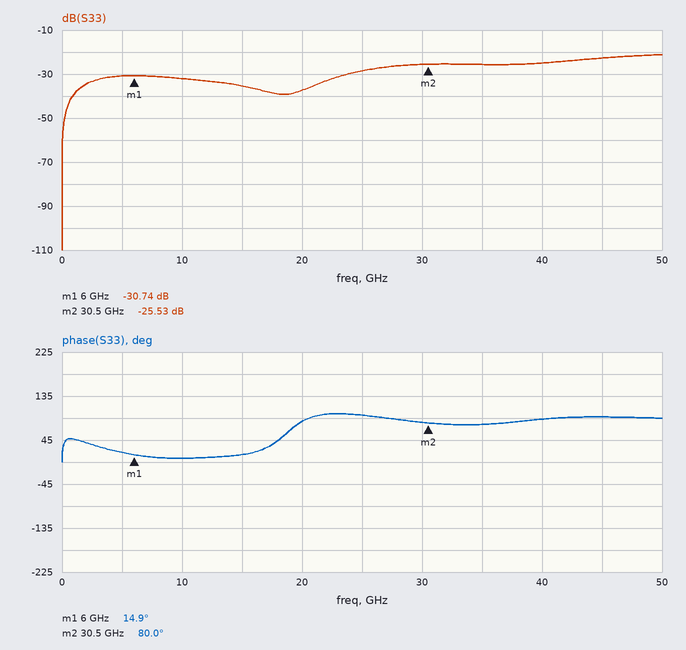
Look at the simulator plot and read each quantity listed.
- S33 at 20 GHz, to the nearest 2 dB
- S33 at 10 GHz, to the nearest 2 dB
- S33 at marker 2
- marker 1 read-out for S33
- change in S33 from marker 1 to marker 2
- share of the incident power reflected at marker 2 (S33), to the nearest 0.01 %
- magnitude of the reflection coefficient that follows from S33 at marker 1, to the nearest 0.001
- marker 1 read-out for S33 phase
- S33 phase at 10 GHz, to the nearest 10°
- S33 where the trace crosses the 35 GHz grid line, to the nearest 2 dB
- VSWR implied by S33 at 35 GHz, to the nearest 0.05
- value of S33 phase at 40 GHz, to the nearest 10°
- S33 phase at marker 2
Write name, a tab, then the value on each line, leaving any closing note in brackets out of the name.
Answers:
S33 at 20 GHz, to the nearest 2 dB	-38 dB
S33 at 10 GHz, to the nearest 2 dB	-32 dB
S33 at marker 2	-25.53 dB
marker 1 read-out for S33	-30.74 dB
change in S33 from marker 1 to marker 2	5.21 dB
share of the incident power reflected at marker 2 (S33), to the nearest 0.01 %	0.28 %
magnitude of the reflection coefficient that follows from S33 at marker 1, to the nearest 0.001	0.029
marker 1 read-out for S33 phase	14.9°
S33 phase at 10 GHz, to the nearest 10°	10°
S33 where the trace crosses the 35 GHz grid line, to the nearest 2 dB	-26 dB
VSWR implied by S33 at 35 GHz, to the nearest 0.05	1.10
value of S33 phase at 40 GHz, to the nearest 10°	90°
S33 phase at marker 2	80.0°
